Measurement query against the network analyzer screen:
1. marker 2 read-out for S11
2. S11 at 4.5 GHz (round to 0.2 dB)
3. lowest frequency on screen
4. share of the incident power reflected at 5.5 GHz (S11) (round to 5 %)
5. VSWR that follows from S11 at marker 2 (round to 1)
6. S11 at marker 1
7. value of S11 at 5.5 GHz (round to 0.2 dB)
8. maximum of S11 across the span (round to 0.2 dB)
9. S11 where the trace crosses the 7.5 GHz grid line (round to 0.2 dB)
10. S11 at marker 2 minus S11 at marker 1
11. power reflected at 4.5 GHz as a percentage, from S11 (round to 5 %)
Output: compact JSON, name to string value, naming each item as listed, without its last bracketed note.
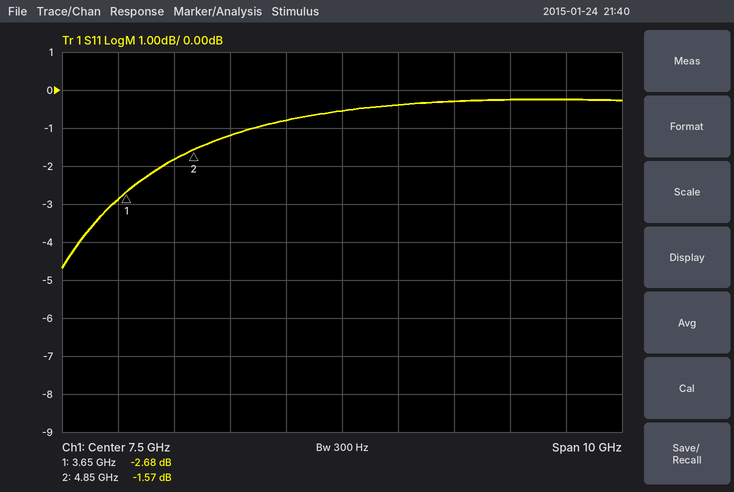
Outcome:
{"marker 2 read-out for S11": "-1.57 dB", "S11 at 4.5 GHz": "-1.8 dB", "lowest frequency on screen": "2.5 GHz", "share of the incident power reflected at 5.5 GHz (S11)": "75 %", "VSWR that follows from S11 at marker 2": "11", "S11 at marker 1": "-2.68 dB", "value of S11 at 5.5 GHz": "-1.2 dB", "maximum of S11 across the span": "-0.2 dB", "S11 where the trace crosses the 7.5 GHz grid line": "-0.6 dB", "S11 at marker 2 minus S11 at marker 1": "1.11 dB", "power reflected at 4.5 GHz as a percentage, from S11": "65 %"}
